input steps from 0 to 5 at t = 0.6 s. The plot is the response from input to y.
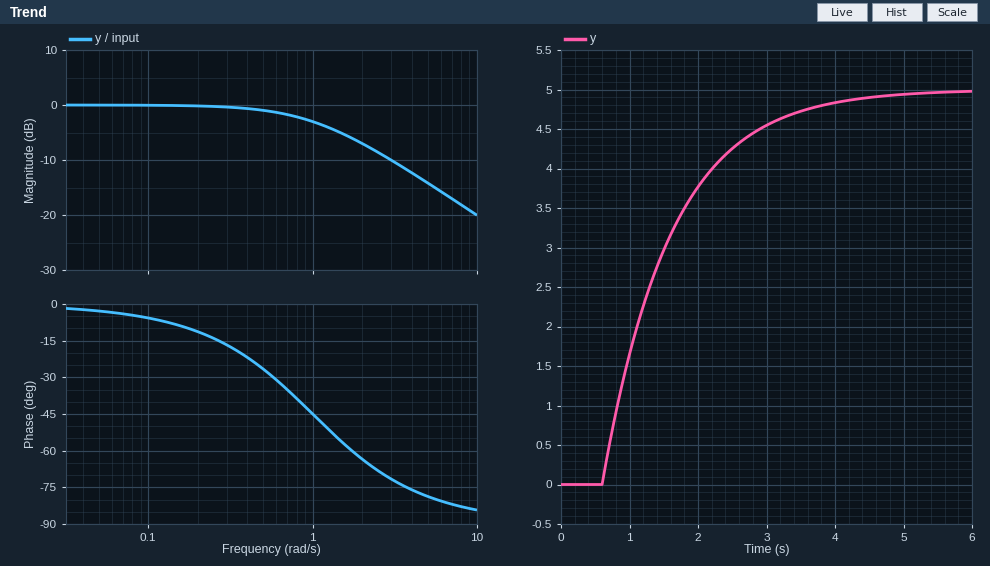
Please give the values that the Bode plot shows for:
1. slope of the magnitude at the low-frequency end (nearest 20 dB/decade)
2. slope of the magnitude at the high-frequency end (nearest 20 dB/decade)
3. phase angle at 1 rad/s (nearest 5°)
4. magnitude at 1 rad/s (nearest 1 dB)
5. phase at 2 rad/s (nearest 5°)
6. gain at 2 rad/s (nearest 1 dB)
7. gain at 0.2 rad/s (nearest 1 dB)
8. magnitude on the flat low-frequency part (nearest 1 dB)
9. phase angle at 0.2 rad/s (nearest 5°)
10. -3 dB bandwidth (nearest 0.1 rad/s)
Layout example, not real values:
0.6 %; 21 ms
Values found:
0 dB/decade; -20 dB/decade; -45°; -3 dB; -65°; -7 dB; 0 dB; 0 dB; -10°; 1.0 rad/s
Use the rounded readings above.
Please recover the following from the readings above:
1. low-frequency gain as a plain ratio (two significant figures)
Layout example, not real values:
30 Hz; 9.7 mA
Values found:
1.0
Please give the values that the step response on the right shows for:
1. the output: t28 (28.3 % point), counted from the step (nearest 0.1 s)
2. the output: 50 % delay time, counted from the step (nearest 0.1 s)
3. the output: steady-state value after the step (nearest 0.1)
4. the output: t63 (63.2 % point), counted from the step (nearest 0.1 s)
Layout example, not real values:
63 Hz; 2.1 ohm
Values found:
0.3 s; 0.7 s; 5.0; 1.0 s
